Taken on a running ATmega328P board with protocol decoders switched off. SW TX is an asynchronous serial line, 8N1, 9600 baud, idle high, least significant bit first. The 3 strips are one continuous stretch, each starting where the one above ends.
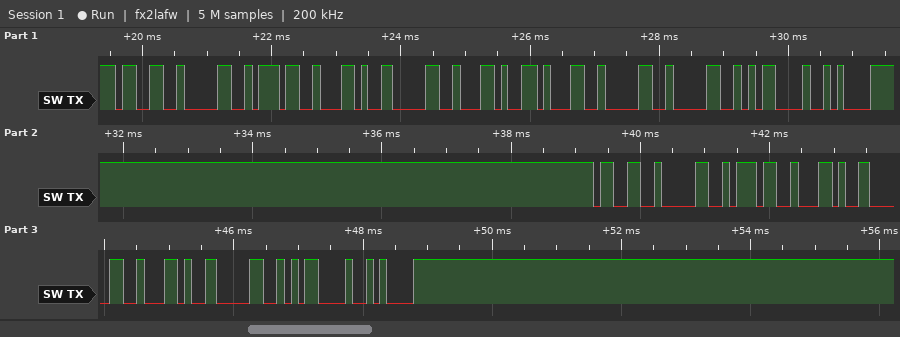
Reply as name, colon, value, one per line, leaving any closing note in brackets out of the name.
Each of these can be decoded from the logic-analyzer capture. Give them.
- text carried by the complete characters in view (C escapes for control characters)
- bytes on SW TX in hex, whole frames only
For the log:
text carried by the complete characters in view: "307,0,100\r\n307,0,0\r\n"
bytes on SW TX in hex, whole frames only: 33 30 37 2C 30 2C 31 30 30 0D 0A 33 30 37 2C 30 2C 30 0D 0A
